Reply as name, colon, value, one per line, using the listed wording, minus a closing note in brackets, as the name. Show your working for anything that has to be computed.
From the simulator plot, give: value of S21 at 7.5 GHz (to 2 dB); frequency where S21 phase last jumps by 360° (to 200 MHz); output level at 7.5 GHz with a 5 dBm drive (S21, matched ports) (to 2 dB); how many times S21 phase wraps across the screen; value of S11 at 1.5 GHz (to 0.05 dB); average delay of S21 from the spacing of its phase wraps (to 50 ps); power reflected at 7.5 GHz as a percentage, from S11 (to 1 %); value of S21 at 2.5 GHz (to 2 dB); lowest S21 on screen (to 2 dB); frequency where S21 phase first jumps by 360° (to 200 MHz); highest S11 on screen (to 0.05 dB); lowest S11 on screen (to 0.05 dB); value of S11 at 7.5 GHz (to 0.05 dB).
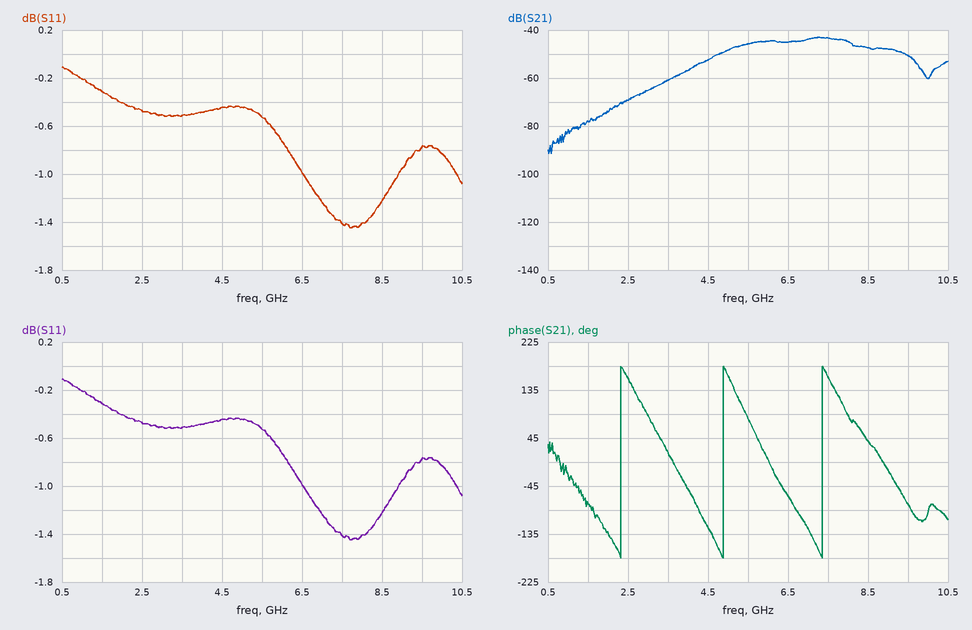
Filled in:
value of S21 at 7.5 GHz: -44 dB
frequency where S21 phase last jumps by 360°: 7.4 GHz
output level at 7.5 GHz with a 5 dBm drive (S21, matched ports): 5 dBm + (-44 dB) = -38 dBm
how many times S21 phase wraps across the screen: 3
value of S11 at 1.5 GHz: -0.30 dB
average delay of S21 from the spacing of its phase wraps: 2 cycles / (7.4 GHz − 2.4 GHz) ≈ 400 ps
power reflected at 7.5 GHz as a percentage, from S11: 10^(-1.4/10) ≈ 72 %
value of S21 at 2.5 GHz: -70 dB
lowest S21 on screen: -92 dB
frequency where S21 phase first jumps by 360°: 2.4 GHz
highest S11 on screen: -0.10 dB
lowest S11 on screen: -1.45 dB
value of S11 at 7.5 GHz: -1.40 dB
